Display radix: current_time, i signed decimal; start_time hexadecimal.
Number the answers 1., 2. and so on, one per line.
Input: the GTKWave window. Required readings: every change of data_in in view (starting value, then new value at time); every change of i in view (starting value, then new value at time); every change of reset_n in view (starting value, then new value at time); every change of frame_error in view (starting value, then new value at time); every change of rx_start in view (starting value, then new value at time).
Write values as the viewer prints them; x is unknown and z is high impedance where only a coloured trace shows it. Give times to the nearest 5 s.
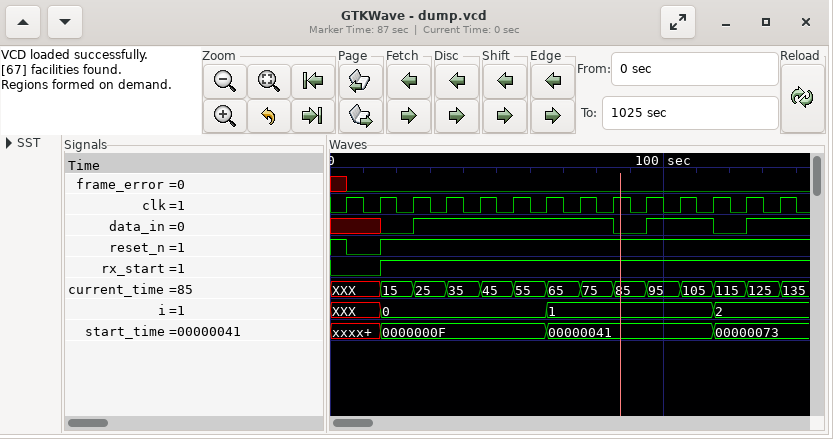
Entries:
1. x, 0 at 15 s, 1 at 25 s, 0 at 85 s, 1 at 95 s, 0 at 115 s, 1 at 125 s
2. XXX, 0 at 15 s, 1 at 65 s, 2 at 115 s
3. 1, 0 at 5 s, 1 at 15 s
4. x, 0 at 5 s
5. 0, 1 at 15 s
